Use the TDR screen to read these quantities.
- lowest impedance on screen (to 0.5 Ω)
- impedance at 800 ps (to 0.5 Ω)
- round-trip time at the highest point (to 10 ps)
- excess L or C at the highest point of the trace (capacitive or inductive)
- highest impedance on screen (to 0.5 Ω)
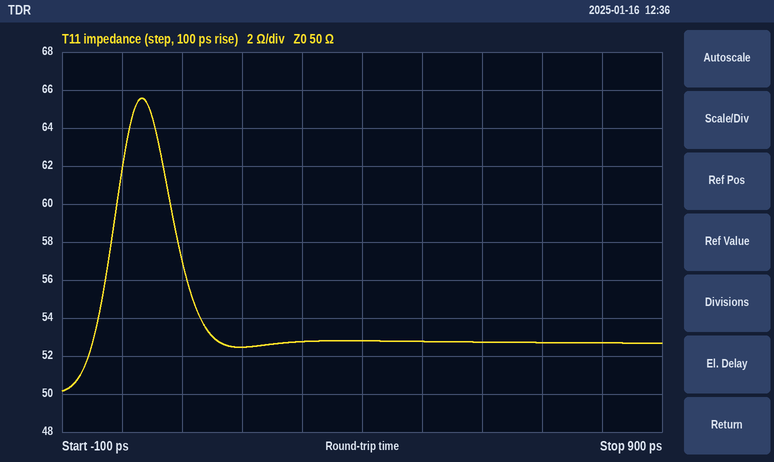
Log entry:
50.0 Ω
52.5 Ω
30 ps
inductive
65.5 Ω
